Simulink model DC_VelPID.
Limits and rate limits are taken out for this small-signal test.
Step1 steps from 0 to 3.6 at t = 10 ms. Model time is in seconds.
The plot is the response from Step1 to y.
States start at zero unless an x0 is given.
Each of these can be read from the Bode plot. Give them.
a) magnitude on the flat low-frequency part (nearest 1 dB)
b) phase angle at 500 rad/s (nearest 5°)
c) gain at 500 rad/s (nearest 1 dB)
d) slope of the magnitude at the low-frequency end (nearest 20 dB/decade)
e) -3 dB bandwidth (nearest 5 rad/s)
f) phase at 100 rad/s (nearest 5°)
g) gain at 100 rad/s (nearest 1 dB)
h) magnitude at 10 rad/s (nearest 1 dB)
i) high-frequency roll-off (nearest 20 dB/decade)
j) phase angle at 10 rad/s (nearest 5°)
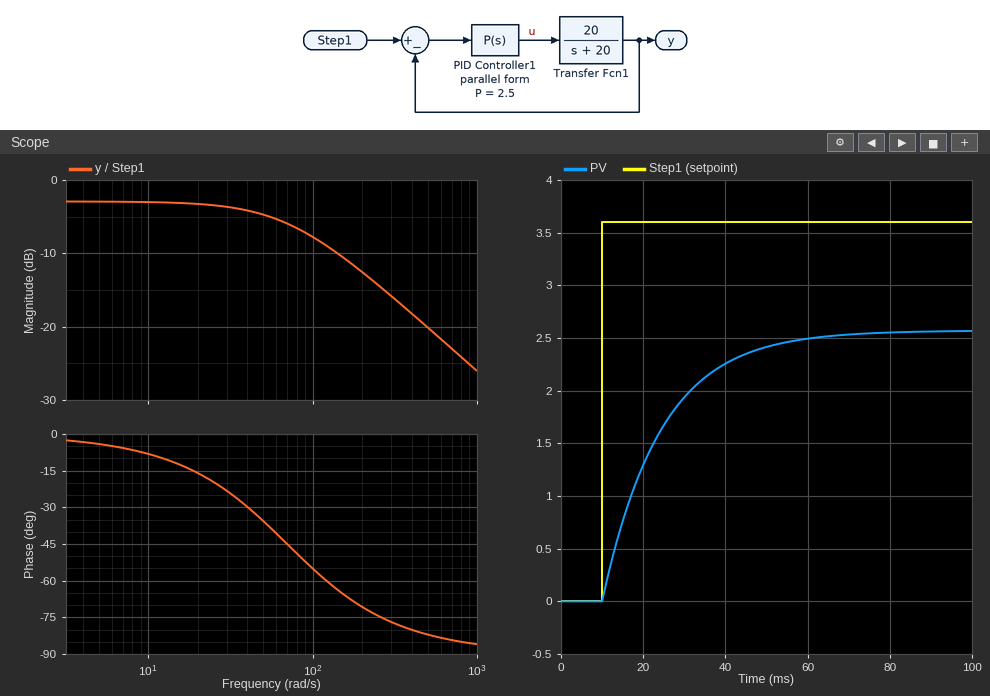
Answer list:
-3 dB
-80°
-20 dB
0 dB/decade
70 rad/s
-55°
-8 dB
-3 dB
-20 dB/decade
-10°
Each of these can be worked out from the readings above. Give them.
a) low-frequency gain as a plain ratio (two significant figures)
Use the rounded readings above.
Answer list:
0.71
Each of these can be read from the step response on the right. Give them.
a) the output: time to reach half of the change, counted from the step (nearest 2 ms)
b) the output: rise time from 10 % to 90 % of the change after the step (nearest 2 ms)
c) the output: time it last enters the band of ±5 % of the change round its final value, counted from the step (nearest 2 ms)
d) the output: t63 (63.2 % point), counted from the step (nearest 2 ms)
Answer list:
10 ms
32 ms
42 ms
14 ms
